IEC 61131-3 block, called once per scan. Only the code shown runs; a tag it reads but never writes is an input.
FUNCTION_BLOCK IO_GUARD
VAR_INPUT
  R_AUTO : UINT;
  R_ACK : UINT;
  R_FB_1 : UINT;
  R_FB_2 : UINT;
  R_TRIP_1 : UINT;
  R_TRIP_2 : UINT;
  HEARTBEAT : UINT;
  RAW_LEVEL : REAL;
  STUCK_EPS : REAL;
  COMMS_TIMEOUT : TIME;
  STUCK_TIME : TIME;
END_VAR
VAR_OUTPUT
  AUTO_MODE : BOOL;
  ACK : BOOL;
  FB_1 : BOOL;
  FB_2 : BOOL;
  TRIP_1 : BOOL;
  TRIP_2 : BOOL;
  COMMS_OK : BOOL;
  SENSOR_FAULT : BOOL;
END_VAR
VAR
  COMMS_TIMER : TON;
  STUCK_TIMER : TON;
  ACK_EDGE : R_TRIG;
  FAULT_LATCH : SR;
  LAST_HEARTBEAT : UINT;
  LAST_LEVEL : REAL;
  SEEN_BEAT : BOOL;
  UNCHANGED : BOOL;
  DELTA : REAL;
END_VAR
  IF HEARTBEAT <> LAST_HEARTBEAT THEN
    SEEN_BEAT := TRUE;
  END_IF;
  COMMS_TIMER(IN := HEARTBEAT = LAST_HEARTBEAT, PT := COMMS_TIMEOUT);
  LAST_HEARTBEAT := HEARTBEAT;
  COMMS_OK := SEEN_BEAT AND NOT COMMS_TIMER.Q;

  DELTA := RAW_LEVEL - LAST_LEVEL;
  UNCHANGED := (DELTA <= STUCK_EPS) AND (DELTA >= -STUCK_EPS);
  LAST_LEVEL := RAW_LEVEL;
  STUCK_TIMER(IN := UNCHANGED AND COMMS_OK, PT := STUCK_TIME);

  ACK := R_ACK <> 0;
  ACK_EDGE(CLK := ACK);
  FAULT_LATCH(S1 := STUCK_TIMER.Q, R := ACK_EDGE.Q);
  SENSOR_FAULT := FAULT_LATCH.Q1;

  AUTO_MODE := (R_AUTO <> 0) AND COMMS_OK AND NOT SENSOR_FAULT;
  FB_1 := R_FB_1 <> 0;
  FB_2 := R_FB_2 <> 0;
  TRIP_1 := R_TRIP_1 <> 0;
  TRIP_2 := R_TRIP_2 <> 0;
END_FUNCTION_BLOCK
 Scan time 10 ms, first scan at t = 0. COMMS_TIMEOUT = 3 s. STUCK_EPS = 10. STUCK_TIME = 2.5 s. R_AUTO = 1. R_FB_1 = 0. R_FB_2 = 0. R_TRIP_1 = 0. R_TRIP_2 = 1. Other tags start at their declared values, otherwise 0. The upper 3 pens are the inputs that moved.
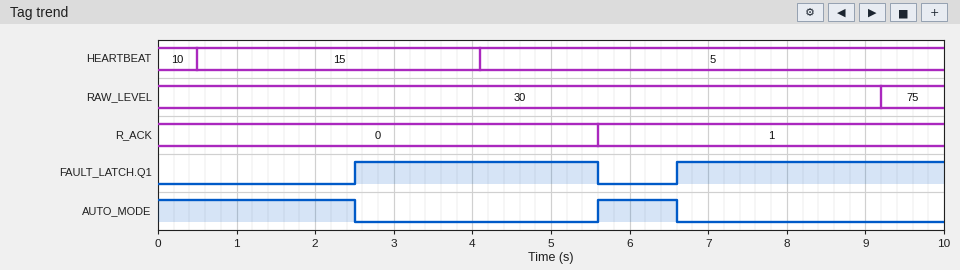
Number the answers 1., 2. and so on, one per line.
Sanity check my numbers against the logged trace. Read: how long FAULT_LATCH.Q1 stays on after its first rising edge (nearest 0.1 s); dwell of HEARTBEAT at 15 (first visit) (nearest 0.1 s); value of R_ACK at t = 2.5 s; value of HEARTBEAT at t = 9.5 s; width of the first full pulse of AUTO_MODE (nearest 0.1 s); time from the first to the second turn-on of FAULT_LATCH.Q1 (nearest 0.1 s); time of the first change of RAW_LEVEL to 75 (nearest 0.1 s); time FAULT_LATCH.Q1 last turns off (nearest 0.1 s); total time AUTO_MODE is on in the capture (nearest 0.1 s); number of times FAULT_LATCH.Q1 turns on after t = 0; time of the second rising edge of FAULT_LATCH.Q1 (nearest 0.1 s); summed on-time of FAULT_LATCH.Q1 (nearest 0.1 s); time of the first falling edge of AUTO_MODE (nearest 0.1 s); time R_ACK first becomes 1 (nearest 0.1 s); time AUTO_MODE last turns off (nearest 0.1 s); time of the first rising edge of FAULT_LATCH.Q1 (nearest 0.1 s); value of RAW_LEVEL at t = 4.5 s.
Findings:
1. 3.1 s
2. 3.6 s
3. 0
4. 5
5. 1.0 s
6. 4.1 s
7. 9.2 s
8. 5.6 s
9. 3.5 s
10. 2
11. 6.6 s
12. 6.5 s
13. 2.5 s
14. 5.6 s
15. 6.6 s
16. 2.5 s
17. 30
